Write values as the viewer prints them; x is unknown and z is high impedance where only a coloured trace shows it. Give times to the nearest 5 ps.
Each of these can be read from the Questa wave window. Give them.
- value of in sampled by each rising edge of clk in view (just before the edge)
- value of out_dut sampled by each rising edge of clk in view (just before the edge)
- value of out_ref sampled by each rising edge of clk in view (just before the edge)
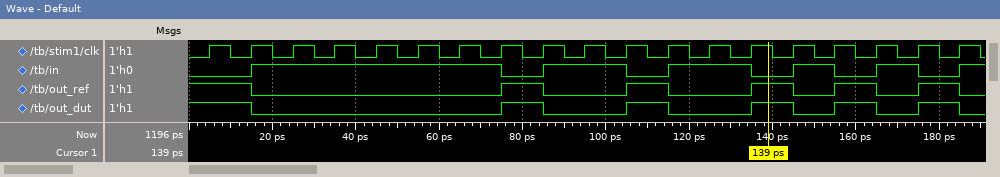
0 0 1 1 1 1 1 1 0 1 1 0 1 1 0 1 0 1 0
1 1 0 0 0 0 0 0 1 0 0 1 0 0 1 0 1 0 1
1 1 0 0 0 0 0 0 1 0 0 1 0 0 1 0 1 0 1
